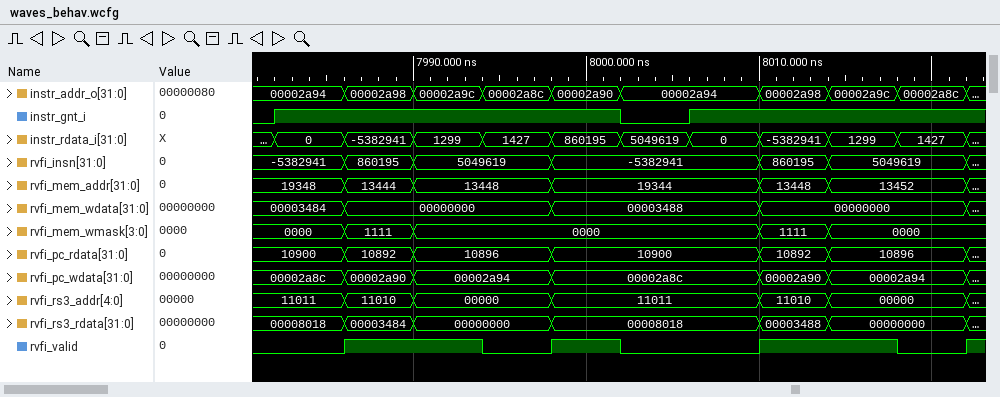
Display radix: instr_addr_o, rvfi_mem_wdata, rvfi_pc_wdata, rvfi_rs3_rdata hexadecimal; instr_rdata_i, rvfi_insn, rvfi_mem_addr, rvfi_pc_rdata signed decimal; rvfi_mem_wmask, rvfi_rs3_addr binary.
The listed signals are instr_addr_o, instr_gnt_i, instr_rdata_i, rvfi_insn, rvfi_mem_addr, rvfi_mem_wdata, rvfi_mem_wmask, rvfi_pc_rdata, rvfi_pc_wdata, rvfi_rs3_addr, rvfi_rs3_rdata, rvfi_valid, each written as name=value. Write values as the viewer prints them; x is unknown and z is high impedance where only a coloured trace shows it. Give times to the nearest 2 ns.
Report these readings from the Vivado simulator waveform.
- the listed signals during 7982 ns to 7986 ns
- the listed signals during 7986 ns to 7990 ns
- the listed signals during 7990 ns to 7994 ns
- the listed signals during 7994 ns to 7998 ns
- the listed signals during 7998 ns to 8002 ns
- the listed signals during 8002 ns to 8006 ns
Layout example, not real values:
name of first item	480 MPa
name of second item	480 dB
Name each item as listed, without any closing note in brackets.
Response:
the listed signals during 7982 ns to 7986 ns	instr_addr_o=00002a94, instr_gnt_i=1, instr_rdata_i=0, rvfi_insn=-5382941, rvfi_mem_addr=19348, rvfi_mem_wdata=00003484, rvfi_mem_wmask=0000, rvfi_pc_rdata=10900, rvfi_pc_wdata=00002a8c, rvfi_rs3_addr=11011, rvfi_rs3_rdata=00008018, rvfi_valid=0
the listed signals during 7986 ns to 7990 ns	instr_addr_o=00002a98, instr_gnt_i=1, instr_rdata_i=-5382941, rvfi_insn=860195, rvfi_mem_addr=13444, rvfi_mem_wdata=00000000, rvfi_mem_wmask=1111, rvfi_pc_rdata=10892, rvfi_pc_wdata=00002a90, rvfi_rs3_addr=11010, rvfi_rs3_rdata=00003484, rvfi_valid=1
the listed signals during 7990 ns to 7994 ns	instr_addr_o=00002a9c, instr_gnt_i=1, instr_rdata_i=1299, rvfi_insn=5049619, rvfi_mem_addr=13448, rvfi_mem_wdata=00000000, rvfi_mem_wmask=0000, rvfi_pc_rdata=10896, rvfi_pc_wdata=00002a94, rvfi_rs3_addr=00000, rvfi_rs3_rdata=00000000, rvfi_valid=1
the listed signals during 7994 ns to 7998 ns	instr_addr_o=00002a8c, instr_gnt_i=1, instr_rdata_i=1427, rvfi_insn=5049619, rvfi_mem_addr=13448, rvfi_mem_wdata=00000000, rvfi_mem_wmask=0000, rvfi_pc_rdata=10896, rvfi_pc_wdata=00002a94, rvfi_rs3_addr=00000, rvfi_rs3_rdata=00000000, rvfi_valid=0
the listed signals during 7998 ns to 8002 ns	instr_addr_o=00002a90, instr_gnt_i=1, instr_rdata_i=860195, rvfi_insn=-5382941, rvfi_mem_addr=19344, rvfi_mem_wdata=00003488, rvfi_mem_wmask=0000, rvfi_pc_rdata=10900, rvfi_pc_wdata=00002a8c, rvfi_rs3_addr=11011, rvfi_rs3_rdata=00008018, rvfi_valid=1
the listed signals during 8002 ns to 8006 ns	instr_addr_o=00002a94, instr_gnt_i=0, instr_rdata_i=5049619, rvfi_insn=-5382941, rvfi_mem_addr=19344, rvfi_mem_wdata=00003488, rvfi_mem_wmask=0000, rvfi_pc_rdata=10900, rvfi_pc_wdata=00002a8c, rvfi_rs3_addr=11011, rvfi_rs3_rdata=00008018, rvfi_valid=0
